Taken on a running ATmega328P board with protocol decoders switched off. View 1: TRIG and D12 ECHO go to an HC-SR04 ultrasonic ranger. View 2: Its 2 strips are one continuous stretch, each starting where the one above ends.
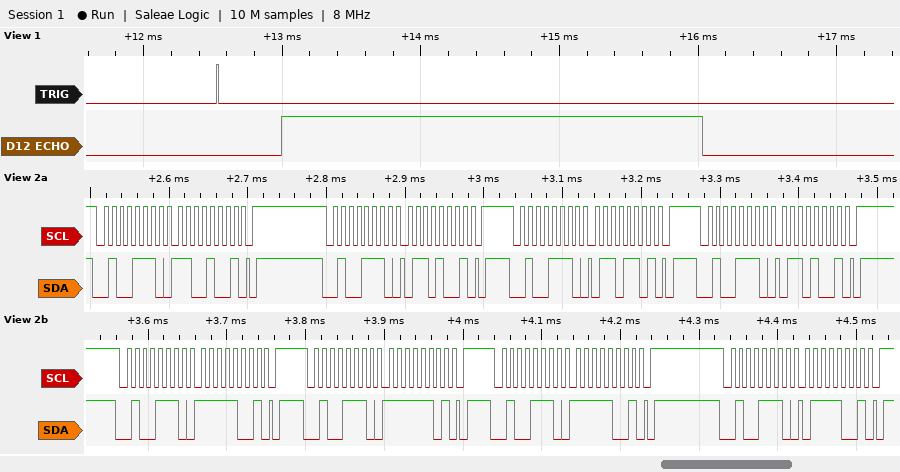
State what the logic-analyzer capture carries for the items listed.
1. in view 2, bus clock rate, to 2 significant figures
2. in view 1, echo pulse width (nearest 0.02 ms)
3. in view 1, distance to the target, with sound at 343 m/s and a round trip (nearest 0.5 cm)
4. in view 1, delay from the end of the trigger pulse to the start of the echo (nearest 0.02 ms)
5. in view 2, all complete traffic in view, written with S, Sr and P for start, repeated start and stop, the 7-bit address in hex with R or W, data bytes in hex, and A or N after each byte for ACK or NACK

100 kHz
3.04 ms
52 cm
0.46 ms
S 27W A C9 A P S 27W A 69 A P S 27W A 6D A P S 27W A 69 A P S 27W A F9 A P S 27W A FD A P S 27W A F9 A P S 27W A 79 A P
